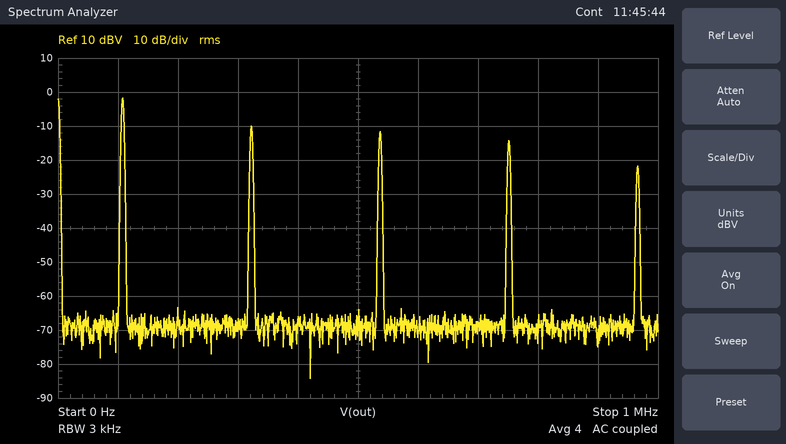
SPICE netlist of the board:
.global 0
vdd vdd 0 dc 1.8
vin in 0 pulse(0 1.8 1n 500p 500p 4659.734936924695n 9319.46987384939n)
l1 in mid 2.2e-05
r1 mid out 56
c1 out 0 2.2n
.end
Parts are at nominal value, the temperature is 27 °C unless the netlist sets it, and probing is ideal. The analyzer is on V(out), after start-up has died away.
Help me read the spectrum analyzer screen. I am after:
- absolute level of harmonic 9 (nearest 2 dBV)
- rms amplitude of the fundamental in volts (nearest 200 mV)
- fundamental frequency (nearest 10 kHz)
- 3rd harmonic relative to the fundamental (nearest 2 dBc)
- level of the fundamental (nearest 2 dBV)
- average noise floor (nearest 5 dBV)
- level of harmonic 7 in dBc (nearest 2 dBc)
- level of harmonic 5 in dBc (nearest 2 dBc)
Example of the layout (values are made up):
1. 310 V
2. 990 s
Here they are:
1. -22 dBV
2. 800 mV
3. 110 kHz
4. -8 dBc
5. -2 dBV
6. -70 dBV
7. -12 dBc
8. -10 dBc
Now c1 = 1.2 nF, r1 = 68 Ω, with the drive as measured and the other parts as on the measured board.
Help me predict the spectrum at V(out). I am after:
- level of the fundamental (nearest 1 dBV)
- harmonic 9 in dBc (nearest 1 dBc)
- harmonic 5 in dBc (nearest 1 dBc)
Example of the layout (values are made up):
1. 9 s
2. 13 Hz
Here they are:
1. -2 dBV
2. -13 dBc
3. -12 dBc
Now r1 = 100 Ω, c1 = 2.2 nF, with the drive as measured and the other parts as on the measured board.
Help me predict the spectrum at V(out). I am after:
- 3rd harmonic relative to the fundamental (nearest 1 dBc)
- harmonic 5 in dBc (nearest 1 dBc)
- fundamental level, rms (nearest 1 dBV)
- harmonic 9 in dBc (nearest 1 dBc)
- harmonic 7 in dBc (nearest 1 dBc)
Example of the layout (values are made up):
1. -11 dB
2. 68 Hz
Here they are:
1. -9 dBc
2. -13 dBc
3. -2 dBV
4. -23 dBc
5. -17 dBc
